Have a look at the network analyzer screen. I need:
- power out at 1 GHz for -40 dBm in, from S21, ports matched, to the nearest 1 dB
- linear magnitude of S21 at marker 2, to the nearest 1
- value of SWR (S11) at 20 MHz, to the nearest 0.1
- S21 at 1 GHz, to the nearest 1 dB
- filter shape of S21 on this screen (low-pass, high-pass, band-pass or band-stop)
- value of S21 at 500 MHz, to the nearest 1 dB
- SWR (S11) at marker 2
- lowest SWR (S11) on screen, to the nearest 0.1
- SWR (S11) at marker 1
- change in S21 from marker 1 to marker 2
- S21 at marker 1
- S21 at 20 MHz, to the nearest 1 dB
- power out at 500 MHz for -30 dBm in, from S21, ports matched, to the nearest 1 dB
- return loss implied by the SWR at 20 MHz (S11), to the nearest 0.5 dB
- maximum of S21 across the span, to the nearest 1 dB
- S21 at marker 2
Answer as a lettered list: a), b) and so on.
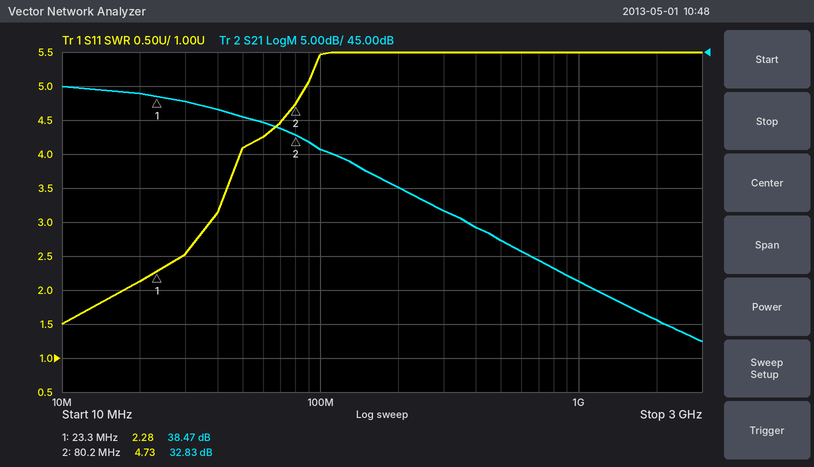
a) -29 dBm
b) 44
c) 2.1
d) 11 dB
e) low-pass
f) 17 dB
g) 4.73
h) 1.5
i) 2.28
j) -5.64 dB
k) 38.47 dB
l) 39 dB
m) -13 dBm
n) 9.0 dB
o) 40 dB
p) 32.83 dB
